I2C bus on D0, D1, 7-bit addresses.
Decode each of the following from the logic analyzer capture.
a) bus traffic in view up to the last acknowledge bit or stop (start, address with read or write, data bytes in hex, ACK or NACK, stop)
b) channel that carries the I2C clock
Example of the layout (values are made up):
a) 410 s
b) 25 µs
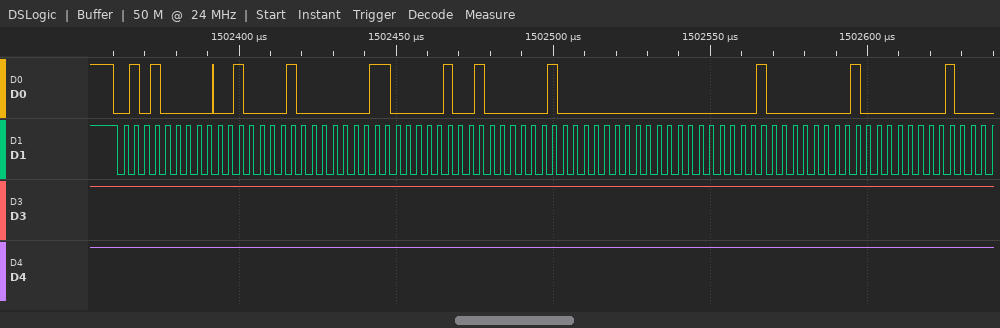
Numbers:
a) start, address 28 write ACK, 21 ACK, 03 ACK, 09 ACK, 04 ACK, 00 ACK, 01 ACK, 01 ACK, 01 ACK
b) D1
